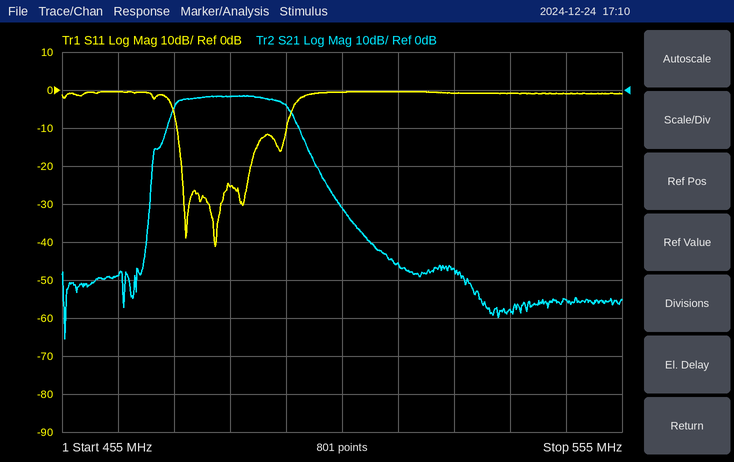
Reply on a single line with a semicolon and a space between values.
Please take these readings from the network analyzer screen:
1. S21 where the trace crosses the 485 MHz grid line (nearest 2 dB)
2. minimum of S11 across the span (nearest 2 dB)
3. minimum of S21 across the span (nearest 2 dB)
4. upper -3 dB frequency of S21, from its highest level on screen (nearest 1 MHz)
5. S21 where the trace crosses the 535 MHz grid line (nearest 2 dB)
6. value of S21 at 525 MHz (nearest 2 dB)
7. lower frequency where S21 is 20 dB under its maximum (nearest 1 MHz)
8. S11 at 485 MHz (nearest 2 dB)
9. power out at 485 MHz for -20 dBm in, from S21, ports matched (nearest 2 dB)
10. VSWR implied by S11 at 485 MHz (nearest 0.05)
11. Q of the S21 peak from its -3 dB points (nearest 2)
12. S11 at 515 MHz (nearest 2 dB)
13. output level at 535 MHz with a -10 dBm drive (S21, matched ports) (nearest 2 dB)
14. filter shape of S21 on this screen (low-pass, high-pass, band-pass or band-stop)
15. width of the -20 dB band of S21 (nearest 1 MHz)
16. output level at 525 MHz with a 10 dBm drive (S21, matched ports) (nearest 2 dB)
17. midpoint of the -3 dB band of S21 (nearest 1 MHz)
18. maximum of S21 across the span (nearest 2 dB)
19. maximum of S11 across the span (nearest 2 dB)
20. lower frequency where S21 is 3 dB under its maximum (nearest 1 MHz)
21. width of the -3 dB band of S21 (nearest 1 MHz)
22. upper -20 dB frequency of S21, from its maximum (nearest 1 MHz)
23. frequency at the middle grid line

-2 dB; -42 dB; -66 dB; 495 MHz; -58 dB; -48 dB; 471 MHz; -26 dB; -22 dBm; 1.10; 24; 0 dB; -68 dBm; band-pass; 30 MHz; -38 dBm; 485 MHz; -2 dB; 0 dB; 475 MHz; 20 MHz; 501 MHz; 505 MHz
